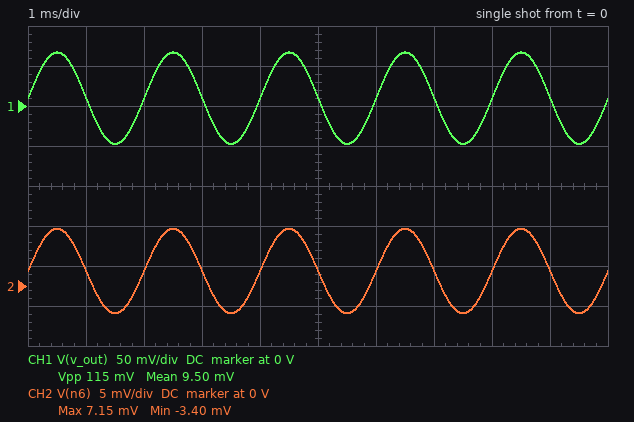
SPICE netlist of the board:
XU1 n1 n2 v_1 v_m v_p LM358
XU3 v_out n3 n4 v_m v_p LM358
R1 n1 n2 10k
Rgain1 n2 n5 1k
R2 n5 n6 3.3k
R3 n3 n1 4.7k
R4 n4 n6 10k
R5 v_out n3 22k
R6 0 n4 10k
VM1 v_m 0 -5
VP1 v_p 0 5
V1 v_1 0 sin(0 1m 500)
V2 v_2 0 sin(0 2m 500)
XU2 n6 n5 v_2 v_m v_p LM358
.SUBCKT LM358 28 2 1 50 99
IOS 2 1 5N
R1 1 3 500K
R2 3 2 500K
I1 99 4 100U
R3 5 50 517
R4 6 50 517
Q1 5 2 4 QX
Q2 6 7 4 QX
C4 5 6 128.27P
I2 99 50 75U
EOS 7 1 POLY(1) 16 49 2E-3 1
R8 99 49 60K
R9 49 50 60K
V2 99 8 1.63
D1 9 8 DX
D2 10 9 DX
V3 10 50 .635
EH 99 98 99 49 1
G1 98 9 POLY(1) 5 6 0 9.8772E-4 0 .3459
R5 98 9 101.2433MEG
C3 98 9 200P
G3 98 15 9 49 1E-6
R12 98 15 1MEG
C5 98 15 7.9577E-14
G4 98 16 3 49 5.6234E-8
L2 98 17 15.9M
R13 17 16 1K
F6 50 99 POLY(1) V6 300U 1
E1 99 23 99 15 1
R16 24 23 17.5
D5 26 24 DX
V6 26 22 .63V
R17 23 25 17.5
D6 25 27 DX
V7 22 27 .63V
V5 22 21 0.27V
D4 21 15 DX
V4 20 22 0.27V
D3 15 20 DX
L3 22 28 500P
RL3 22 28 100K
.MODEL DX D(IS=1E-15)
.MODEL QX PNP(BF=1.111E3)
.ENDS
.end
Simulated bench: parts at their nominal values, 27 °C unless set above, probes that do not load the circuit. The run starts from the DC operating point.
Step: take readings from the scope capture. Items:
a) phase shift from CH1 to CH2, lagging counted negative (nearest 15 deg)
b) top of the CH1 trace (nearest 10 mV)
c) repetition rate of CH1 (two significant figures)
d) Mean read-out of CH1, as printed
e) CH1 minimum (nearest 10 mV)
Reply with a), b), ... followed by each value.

a) 0 deg
b) 70 mV
c) 500 Hz
d) 9.50 mV
e) -50 mV
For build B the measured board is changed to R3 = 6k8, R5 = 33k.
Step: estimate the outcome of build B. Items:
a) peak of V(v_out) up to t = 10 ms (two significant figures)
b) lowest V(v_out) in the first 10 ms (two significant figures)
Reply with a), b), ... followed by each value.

a) 69 mV
b) -50 mV
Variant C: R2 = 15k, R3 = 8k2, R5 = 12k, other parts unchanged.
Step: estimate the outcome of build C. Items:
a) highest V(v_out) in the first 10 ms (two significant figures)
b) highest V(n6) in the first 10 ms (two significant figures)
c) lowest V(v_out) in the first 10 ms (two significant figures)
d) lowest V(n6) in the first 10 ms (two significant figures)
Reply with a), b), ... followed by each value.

a) 39 mV
b) 18 mV
c) -30 mV
d) -16 mV
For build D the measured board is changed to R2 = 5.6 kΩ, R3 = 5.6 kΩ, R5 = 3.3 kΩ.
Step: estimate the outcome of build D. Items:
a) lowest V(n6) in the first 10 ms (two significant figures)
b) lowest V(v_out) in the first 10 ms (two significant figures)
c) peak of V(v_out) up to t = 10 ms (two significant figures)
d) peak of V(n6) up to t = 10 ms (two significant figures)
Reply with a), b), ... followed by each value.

a) -5.8 mV
b) -7.4 mV
c) 15 mV
d) 9.4 mV
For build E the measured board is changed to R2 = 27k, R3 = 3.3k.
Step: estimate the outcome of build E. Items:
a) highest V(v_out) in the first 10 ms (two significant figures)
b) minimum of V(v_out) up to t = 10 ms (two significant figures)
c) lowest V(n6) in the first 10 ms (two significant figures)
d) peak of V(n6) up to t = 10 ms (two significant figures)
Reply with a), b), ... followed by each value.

a) 180 mV
b) -160 mV
c) -28 mV
d) 30 mV
